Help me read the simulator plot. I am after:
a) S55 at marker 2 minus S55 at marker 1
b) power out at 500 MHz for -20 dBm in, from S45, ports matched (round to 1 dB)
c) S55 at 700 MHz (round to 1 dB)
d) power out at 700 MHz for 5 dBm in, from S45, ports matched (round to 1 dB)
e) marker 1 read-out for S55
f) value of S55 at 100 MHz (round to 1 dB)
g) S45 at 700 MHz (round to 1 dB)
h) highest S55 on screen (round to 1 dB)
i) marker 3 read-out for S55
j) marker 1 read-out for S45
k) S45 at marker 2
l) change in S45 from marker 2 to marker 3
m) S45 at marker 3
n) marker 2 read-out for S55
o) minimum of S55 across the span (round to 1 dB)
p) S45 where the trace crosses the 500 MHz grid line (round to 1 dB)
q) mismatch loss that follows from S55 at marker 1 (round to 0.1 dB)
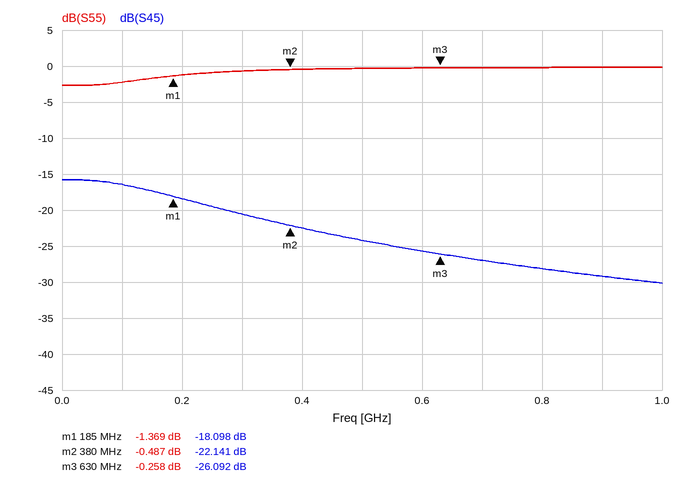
0.882 dB
-44 dBm
0 dB
-22 dBm
-1.369 dB
-2 dB
-27 dB
0 dB
-0.258 dB
-18.098 dB
-22.141 dB
-3.951 dB
-26.092 dB
-0.487 dB
-3 dB
-24 dB
5.7 dB
